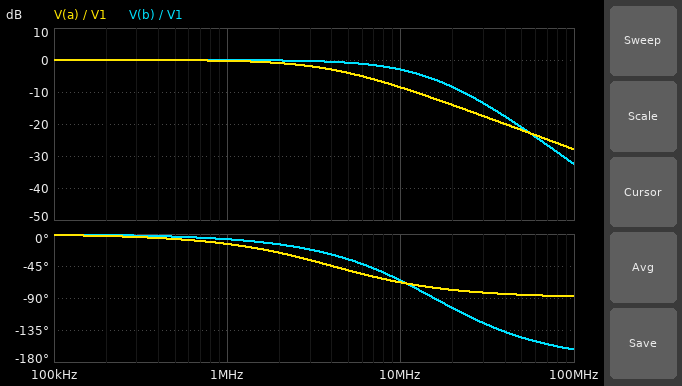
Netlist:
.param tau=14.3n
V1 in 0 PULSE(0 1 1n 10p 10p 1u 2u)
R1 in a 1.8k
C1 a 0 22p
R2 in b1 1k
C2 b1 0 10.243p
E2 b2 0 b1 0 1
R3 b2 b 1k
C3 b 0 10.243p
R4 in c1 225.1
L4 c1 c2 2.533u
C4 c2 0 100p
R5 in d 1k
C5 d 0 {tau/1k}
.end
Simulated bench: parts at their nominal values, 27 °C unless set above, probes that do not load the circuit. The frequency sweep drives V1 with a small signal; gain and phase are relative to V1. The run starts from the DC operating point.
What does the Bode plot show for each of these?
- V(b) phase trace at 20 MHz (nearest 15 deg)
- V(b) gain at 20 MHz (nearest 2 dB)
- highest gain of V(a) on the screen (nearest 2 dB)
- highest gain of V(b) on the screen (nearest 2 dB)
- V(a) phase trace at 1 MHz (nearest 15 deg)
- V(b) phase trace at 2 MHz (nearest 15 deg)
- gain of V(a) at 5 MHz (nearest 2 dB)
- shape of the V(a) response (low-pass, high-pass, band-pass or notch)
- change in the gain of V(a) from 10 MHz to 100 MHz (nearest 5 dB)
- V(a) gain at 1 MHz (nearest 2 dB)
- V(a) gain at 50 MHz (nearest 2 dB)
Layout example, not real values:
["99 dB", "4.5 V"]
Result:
["-105 deg", "-8 dB", "0 dB", "0 dB", "-15 deg", "-15 deg", "-4 dB", "low-pass", "-20 dB", "0 dB", "-22 dB"]
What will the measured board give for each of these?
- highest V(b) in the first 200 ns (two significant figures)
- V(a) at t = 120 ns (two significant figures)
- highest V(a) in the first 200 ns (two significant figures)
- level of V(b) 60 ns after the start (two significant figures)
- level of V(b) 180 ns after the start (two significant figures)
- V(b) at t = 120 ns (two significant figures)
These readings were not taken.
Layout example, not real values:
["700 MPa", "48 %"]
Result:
["1.0 V", "950 mV", "990 mV", "980 mV", "1.0 V", "1.0 V"]
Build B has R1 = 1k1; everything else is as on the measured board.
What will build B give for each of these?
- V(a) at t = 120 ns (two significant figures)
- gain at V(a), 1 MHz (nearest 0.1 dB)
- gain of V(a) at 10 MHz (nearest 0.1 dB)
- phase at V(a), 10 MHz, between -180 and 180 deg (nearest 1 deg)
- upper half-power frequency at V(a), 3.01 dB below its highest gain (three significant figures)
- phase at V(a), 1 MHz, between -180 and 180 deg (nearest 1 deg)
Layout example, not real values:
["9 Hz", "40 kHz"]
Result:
["990 mV", "-0.1 dB", "-5.2 dB", "-57 deg", "6.58 MHz", "-9 deg"]
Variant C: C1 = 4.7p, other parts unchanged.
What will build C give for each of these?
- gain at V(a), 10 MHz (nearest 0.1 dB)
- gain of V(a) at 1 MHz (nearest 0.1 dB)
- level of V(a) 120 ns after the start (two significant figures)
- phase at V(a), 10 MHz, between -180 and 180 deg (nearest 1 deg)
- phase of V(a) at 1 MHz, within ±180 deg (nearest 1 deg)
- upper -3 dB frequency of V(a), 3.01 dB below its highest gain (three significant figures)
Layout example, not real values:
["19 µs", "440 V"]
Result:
["-1.1 dB", "0 dB", "1.0 V", "-28 deg", "-3 deg", "18.8 MHz"]
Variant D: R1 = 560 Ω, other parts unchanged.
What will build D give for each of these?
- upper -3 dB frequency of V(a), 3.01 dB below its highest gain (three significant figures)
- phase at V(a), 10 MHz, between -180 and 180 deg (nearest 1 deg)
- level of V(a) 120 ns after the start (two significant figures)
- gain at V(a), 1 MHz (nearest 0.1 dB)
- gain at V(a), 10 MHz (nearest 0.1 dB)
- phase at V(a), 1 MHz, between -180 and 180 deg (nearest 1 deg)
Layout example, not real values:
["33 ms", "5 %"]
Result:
["12.9 MHz", "-38 deg", "1.0 V", "0 dB", "-2.0 dB", "-4 deg"]
